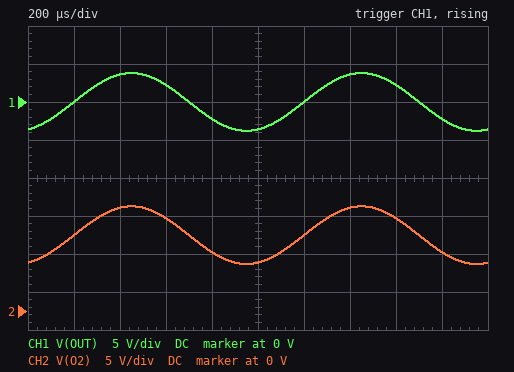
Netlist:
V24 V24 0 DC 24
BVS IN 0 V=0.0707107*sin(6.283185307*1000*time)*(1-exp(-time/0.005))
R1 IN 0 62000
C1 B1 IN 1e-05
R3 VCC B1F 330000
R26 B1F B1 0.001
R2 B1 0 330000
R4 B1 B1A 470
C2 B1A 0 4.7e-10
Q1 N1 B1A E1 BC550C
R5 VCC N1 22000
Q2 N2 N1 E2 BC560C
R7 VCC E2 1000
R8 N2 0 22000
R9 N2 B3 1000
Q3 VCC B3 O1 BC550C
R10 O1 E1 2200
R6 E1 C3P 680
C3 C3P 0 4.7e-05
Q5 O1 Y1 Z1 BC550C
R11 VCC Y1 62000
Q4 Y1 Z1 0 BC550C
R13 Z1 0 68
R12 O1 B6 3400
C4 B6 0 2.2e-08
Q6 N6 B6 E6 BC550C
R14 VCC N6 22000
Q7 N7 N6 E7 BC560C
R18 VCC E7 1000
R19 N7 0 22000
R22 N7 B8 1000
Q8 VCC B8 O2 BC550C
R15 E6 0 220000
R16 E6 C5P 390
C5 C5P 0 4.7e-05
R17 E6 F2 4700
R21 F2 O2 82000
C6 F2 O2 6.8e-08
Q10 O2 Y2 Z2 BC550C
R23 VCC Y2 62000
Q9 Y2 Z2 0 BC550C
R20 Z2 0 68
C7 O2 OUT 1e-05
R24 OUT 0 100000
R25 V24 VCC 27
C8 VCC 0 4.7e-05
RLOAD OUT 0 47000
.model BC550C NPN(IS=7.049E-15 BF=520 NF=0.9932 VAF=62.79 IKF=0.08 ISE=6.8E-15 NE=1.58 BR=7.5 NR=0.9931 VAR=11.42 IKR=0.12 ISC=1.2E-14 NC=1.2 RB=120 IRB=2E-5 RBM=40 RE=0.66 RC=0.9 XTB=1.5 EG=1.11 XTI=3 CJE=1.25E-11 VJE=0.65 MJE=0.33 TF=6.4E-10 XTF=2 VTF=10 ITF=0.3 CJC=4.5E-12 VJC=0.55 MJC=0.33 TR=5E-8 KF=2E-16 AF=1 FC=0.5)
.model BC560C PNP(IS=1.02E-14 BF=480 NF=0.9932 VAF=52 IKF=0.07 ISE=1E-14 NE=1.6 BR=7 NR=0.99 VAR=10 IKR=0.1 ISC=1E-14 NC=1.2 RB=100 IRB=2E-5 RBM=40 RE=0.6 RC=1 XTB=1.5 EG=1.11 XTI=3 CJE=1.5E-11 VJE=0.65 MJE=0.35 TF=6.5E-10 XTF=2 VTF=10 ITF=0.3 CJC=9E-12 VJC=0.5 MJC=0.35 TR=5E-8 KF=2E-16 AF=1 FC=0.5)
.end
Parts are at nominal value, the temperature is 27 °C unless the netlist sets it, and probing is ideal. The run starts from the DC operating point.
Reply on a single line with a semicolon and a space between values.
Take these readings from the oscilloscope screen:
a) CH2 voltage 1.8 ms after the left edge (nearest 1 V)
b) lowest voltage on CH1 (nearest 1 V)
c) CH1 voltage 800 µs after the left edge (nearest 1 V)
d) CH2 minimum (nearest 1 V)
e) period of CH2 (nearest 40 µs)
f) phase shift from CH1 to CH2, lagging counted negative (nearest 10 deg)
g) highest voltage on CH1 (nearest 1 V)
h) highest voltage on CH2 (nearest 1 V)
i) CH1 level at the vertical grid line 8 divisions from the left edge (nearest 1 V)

8 V; -4 V; -2 V; 6 V; 1.00 ms; 0 deg; 4 V; 14 V; 2 V
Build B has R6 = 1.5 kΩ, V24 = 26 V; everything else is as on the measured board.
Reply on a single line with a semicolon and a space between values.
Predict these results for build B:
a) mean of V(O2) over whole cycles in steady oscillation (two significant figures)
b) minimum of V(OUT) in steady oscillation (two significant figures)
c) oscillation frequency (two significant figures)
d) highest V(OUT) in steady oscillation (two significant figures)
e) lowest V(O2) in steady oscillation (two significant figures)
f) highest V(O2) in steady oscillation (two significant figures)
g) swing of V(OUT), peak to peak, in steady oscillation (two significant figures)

11 V; -2.2 V; 1.0 kHz; 2.2 V; 8.9 V; 13 V; 4.4 V
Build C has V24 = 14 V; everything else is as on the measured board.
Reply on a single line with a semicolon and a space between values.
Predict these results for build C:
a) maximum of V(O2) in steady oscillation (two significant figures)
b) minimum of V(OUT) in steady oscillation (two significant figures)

8.0 V; -3.7 V
